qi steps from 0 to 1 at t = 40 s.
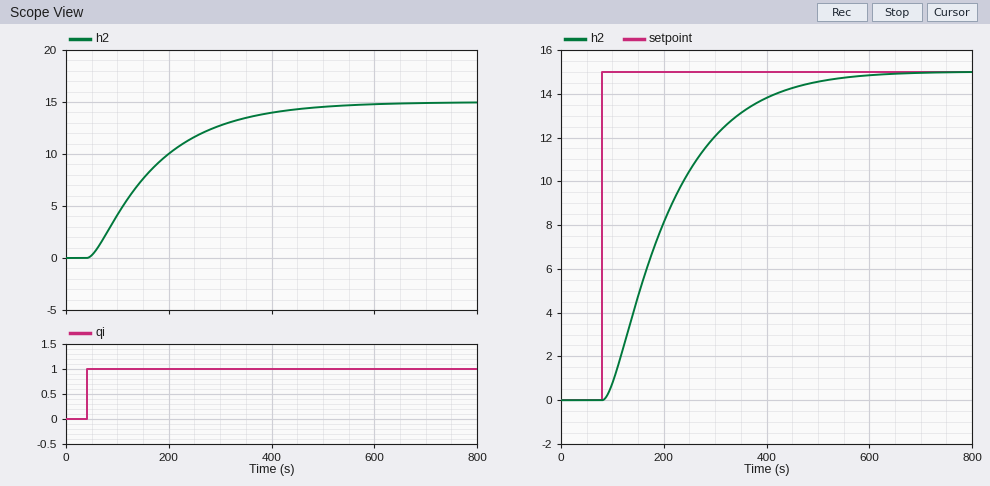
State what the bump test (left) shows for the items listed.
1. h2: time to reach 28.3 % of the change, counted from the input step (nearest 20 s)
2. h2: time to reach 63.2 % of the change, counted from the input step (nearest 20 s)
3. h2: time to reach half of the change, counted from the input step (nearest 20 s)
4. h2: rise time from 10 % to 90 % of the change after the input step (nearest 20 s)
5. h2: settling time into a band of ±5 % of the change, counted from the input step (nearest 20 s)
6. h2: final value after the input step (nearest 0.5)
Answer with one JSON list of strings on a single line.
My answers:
["60 s", "140 s", "100 s", "280 s", "400 s", "15.0"]
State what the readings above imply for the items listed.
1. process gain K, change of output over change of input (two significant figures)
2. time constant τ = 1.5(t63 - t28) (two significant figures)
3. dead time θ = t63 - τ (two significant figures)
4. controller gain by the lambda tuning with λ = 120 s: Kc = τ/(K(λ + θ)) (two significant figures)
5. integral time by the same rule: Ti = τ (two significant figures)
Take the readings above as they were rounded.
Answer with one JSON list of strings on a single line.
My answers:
["15", "120 s", "20 s", "0.057", "120 s"]
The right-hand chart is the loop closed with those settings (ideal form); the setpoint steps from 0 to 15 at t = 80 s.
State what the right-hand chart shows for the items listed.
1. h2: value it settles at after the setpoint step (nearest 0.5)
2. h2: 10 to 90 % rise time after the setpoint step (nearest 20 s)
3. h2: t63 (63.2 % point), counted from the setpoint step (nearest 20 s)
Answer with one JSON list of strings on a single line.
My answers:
["15.0", "260 s", "140 s"]
